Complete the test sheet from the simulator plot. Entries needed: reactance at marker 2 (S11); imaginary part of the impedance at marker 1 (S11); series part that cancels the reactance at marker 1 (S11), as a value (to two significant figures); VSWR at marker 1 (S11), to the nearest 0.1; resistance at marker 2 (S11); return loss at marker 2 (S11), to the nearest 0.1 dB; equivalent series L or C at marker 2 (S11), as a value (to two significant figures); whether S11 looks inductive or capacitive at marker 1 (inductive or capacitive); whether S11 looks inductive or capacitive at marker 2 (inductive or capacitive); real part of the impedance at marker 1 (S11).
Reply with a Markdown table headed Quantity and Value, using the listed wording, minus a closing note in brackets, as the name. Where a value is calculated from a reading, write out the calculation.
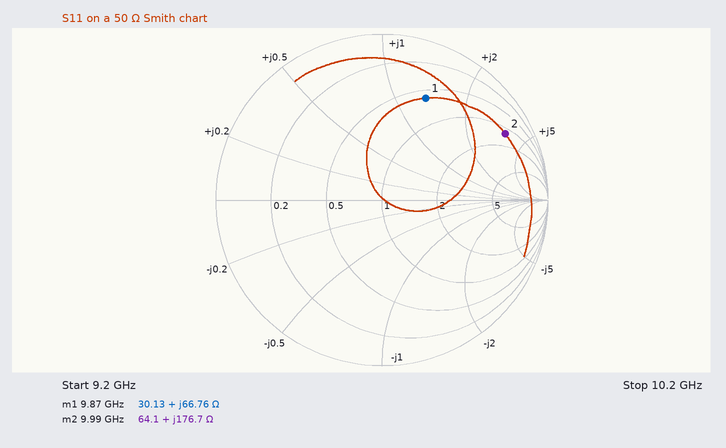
| Quantity | Value |
|---|---|
| reactance at marker 2 | +176.7 Ω |
| imaginary part of the impedance at marker 1 | +66.76 Ω |
| series part that cancels the reactance at marker 1 (S11), as a value | C = 1/(2π × 9.87 GHz × 66.76 Ω) ≈ 242 fF, so 240 fF to two significant figures |
| VSWR at marker 1 (S11), to the nearest 0.1 | 5.0 |
| resistance at marker 2 | 64.1 Ω |
| return loss at marker 2 (S11), to the nearest 0.1 dB | 1.5 dB |
| equivalent series L or C at marker 2 (S11), as a value | L = 176.7 Ω/(2π × 9.99 GHz) ≈ 2.8 nH |
| whether S11 looks inductive or capacitive at marker 1 | inductive |
| whether S11 looks inductive or capacitive at marker 2 | inductive |
| real part of the impedance at marker 1 | 30.13 Ω |
